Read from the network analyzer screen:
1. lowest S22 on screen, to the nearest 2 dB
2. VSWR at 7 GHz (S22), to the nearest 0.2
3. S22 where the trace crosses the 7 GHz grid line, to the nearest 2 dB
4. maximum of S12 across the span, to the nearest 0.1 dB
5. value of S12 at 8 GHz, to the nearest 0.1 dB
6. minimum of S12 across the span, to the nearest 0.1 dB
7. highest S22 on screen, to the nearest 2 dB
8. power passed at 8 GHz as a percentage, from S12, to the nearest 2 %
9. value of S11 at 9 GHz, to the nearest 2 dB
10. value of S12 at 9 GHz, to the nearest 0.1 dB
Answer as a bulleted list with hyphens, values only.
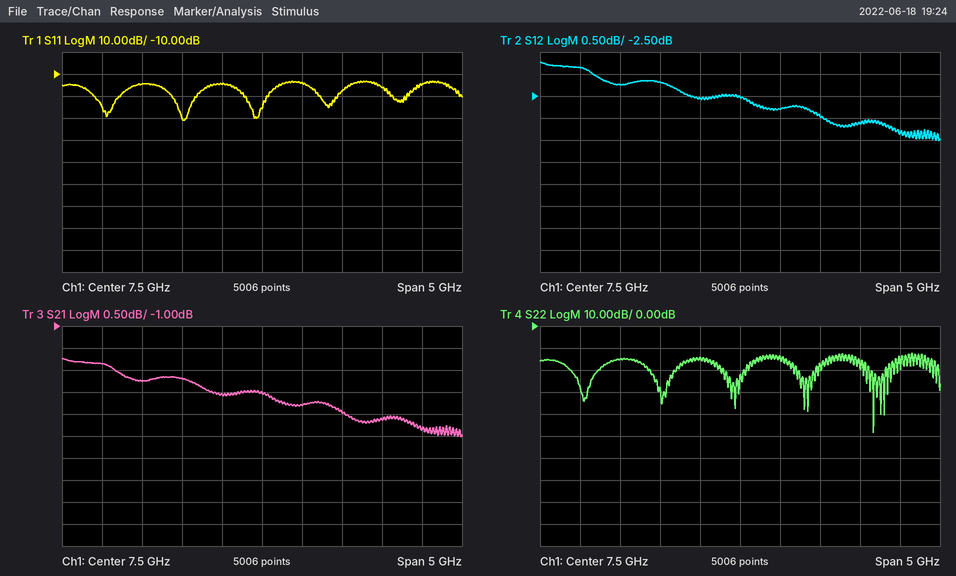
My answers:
- -48 dB
- 1.4
- -14 dB
- -1.7 dB
- -2.8 dB
- -3.5 dB
- -12 dB
- 52 %
- -16 dB
- -3.1 dB
